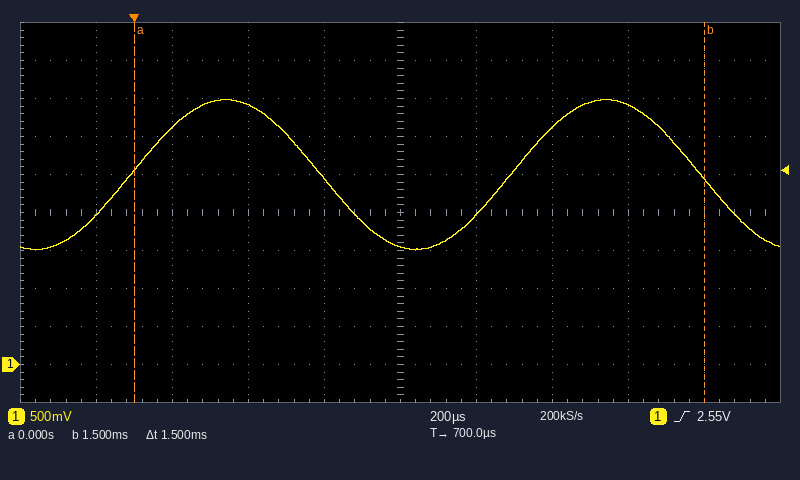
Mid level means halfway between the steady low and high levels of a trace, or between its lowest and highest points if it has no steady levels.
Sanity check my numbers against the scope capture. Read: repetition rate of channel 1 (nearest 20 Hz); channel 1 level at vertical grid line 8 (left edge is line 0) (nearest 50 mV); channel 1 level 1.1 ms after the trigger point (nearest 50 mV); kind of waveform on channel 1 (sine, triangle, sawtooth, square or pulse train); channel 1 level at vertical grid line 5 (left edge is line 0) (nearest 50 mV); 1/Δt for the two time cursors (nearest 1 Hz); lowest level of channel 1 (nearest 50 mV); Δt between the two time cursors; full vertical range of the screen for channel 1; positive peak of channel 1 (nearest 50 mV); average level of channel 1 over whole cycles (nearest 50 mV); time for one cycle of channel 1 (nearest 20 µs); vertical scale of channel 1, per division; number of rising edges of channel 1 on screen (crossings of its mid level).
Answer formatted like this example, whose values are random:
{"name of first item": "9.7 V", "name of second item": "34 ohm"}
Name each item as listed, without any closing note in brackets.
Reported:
{"repetition rate of channel 1": "1.00 kHz", "channel 1 level at vertical grid line 8 (left edge is line 0)": "3.40 V", "channel 1 level 1.1 ms after the trigger point": "3.10 V", "kind of waveform on channel 1": "sine", "channel 1 level at vertical grid line 5 (left edge is line 0)": "1.55 V", "1/Δt for the two time cursors": "667 Hz", "lowest level of channel 1": "1.50 V", "Δt between the two time cursors": "1.5 ms", "full vertical range of the screen for channel 1": "5 V", "positive peak of channel 1": "3.50 V", "average level of channel 1 over whole cycles": "2.50 V", "time for one cycle of channel 1": "1.00 ms", "vertical scale of channel 1, per division": "500 mV", "number of rising edges of channel 1 on screen": "2"}
